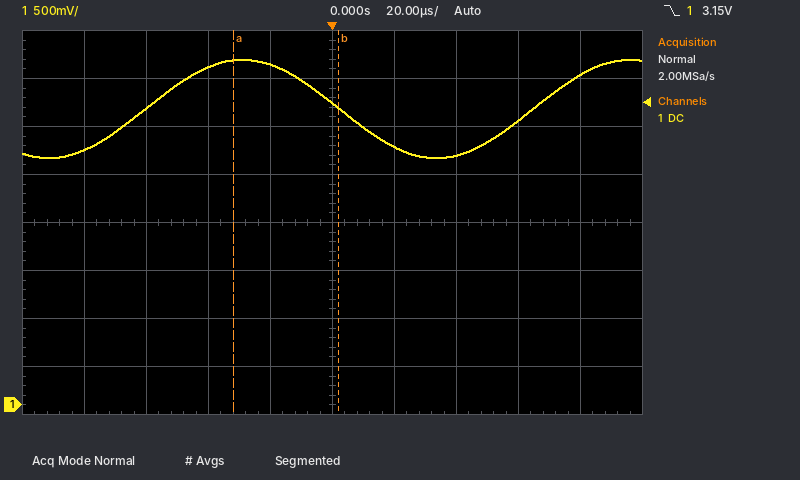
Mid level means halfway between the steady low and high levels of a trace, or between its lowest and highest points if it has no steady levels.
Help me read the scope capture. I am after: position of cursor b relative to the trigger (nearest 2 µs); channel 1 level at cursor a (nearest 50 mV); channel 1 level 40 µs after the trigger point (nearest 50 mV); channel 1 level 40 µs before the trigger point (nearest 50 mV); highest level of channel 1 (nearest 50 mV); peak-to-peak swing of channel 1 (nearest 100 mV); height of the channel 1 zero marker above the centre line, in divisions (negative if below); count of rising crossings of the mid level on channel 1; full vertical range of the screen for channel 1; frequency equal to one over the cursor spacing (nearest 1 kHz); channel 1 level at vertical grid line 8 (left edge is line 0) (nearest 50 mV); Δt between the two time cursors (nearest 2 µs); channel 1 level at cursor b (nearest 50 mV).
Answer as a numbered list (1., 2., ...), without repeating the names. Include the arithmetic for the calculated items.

1. +2 µs
2. 3.60 V
3. 2.60 V
4. 3.50 V
5. 3.60 V
6. 1.00 V
7. -3.8 div
8. 2
9. 4 V
10. 1 / 34 µs ≈ 29 kHz
11. 2.95 V
12. 34 µs
13. 3.10 V
